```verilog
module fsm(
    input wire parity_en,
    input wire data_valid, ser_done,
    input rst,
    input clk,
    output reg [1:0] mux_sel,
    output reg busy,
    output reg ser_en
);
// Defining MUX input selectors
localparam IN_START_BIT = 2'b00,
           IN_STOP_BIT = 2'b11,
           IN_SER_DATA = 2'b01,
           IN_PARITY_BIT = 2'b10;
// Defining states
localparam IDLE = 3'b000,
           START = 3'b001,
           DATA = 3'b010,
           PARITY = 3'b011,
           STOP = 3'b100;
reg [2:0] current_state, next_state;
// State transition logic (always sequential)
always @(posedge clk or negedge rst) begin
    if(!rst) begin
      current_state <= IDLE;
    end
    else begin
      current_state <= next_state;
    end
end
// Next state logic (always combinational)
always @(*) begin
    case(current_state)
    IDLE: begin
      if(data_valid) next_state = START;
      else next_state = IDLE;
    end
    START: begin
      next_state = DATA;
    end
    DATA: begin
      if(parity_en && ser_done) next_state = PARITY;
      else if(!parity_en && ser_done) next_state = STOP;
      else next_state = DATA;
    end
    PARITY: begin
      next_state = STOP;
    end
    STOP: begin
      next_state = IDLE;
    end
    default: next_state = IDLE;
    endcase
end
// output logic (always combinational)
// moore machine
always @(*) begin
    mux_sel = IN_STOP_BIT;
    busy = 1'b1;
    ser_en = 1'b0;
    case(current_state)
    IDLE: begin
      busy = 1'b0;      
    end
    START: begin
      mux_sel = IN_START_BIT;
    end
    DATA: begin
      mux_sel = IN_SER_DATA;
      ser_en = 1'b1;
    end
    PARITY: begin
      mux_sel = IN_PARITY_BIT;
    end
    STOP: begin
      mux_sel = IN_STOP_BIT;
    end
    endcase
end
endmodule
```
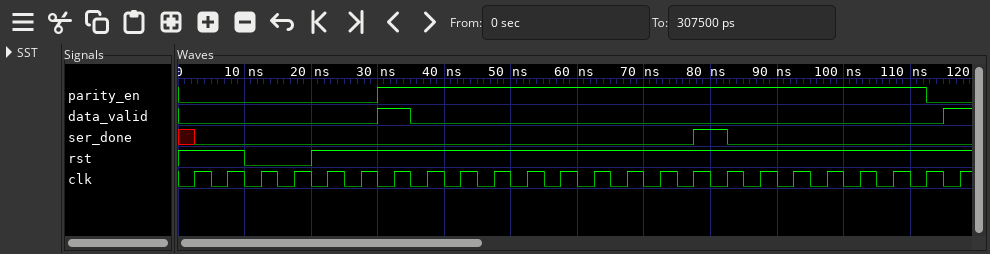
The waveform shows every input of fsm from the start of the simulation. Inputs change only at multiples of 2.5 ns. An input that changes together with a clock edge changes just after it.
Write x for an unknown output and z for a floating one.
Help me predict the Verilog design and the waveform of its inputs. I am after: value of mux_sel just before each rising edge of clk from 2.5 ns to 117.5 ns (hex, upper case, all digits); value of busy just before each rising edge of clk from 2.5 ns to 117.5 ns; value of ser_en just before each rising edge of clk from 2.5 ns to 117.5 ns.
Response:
x, 3, 3, 3, 3, 3, 3, 0, 1, 1, 1, 1, 1, 1, 1, 1, 1, 2, 3, 3, 3, 3, 3, 3
x 0 0 0 0 0 0 1 1 1 1 1 1 1 1 1 1 1 1 0 0 0 0 0
x 0 0 0 0 0 0 0 1 1 1 1 1 1 1 1 1 0 0 0 0 0 0 0
